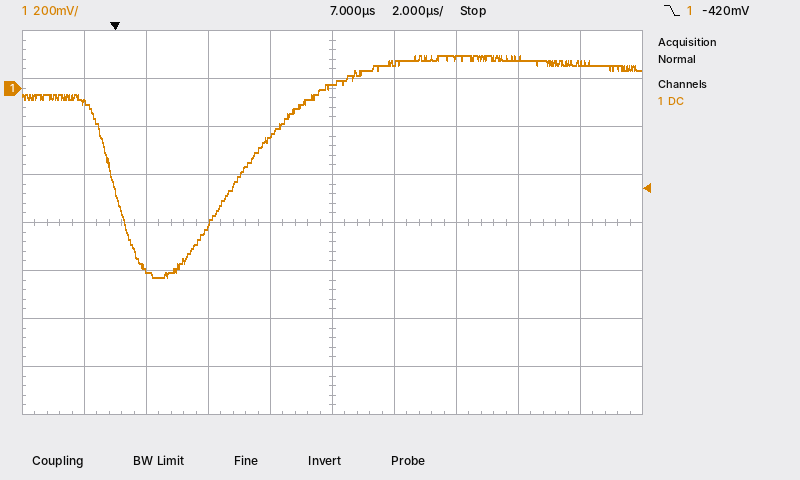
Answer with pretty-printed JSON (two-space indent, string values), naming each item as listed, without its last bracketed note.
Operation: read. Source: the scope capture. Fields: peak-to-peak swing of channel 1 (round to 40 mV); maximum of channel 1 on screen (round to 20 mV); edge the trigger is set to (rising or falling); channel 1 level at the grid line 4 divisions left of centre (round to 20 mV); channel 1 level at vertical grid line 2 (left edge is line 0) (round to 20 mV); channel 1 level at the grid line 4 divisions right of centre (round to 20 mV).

{
  "peak-to-peak swing of channel 1": "920 mV",
  "maximum of channel 1 on screen": "140 mV",
  "edge the trigger is set to": "falling",
  "channel 1 level at the grid line 4 divisions left of centre": "-60 mV",
  "channel 1 level at vertical grid line 2 (left edge is line 0)": "-760 mV",
  "channel 1 level at the grid line 4 divisions right of centre": "100 mV"
}
